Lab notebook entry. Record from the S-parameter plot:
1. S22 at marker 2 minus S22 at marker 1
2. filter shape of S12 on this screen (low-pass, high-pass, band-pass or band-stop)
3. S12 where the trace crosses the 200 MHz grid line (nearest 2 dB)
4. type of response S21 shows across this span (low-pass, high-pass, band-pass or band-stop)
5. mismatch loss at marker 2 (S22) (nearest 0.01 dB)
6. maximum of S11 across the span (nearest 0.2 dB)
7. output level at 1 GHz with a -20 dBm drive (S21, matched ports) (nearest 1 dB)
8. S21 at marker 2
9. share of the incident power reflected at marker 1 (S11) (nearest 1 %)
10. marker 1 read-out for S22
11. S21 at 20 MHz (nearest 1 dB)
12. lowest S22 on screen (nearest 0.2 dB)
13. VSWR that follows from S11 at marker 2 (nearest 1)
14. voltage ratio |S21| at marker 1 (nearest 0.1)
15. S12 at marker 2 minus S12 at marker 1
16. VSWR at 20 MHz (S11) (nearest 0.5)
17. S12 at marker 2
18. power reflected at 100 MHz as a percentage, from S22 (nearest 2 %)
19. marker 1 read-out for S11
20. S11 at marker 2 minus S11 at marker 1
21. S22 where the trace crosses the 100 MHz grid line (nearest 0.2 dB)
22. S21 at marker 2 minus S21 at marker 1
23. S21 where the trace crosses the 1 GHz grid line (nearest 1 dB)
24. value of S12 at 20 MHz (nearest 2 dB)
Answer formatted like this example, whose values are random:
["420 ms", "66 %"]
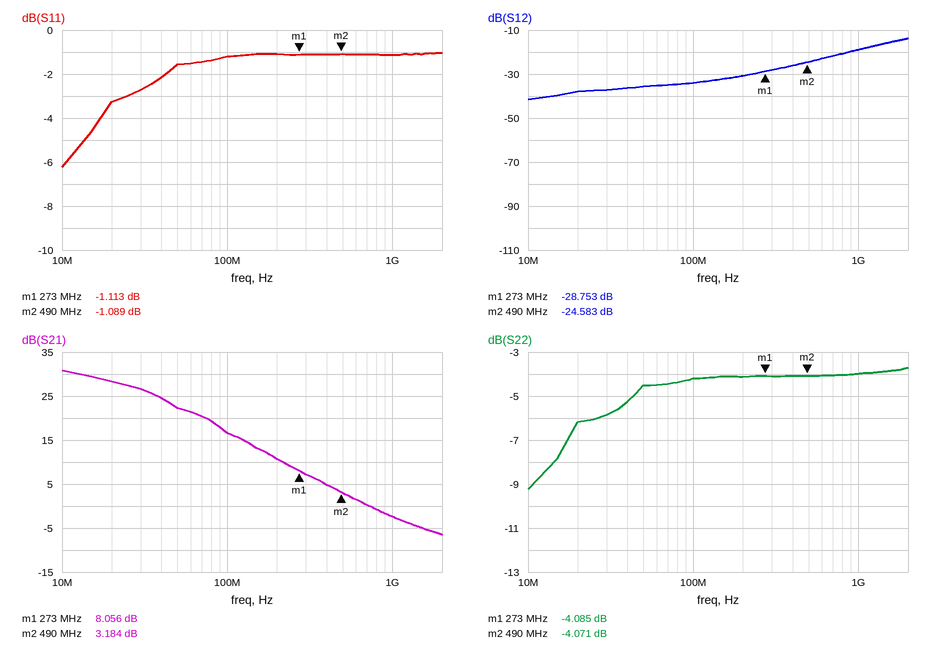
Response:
["0.014 dB", "high-pass", "-30 dB", "low-pass", "2.16 dB", "-1.0 dB", "-22 dBm", "3.184 dB", "77 %", "-4.085 dB", "28 dB", "-9.2 dB", "16", "2.5", "4.170 dB", "5.5", "-24.583 dB", "38 %", "-1.113 dB", "0.024 dB", "-4.2 dB", "-4.872 dB", "-2 dB", "-38 dB"]
